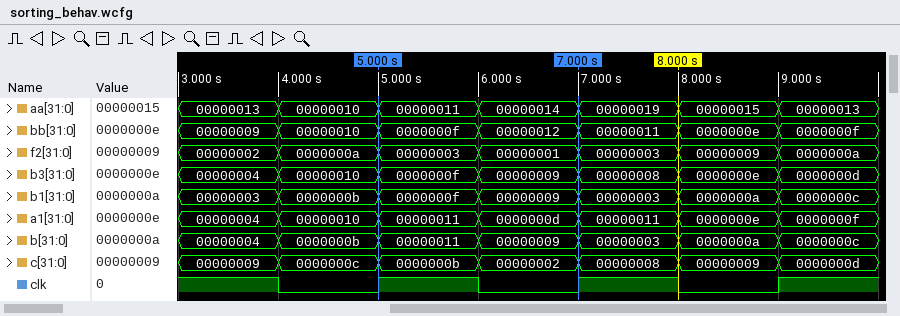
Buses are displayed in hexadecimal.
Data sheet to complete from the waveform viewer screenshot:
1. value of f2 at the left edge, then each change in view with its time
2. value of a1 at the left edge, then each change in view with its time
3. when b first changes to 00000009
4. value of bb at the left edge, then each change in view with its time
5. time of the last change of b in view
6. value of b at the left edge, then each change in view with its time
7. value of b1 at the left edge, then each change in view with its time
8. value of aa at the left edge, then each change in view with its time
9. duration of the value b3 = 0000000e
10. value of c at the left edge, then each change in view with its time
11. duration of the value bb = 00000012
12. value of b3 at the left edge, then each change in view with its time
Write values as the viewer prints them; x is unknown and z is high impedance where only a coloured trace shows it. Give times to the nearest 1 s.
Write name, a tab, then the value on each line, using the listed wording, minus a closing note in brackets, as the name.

value of f2 at the left edge, then each change in view with its time	00000002, 0000000a at 4 s, 00000003 at 5 s, 00000001 at 6 s, 00000003 at 7 s, 00000009 at 8 s, 0000000a at 9 s
value of a1 at the left edge, then each change in view with its time	00000004, 00000010 at 4 s, 00000011 at 5 s, 0000000d at 6 s, 00000011 at 7 s, 0000000e at 8 s, 0000000f at 9 s
when b first changes to 00000009	6 s
value of bb at the left edge, then each change in view with its time	00000009, 00000010 at 4 s, 0000000f at 5 s, 00000012 at 6 s, 00000011 at 7 s, 0000000e at 8 s, 0000000f at 9 s
time of the last change of b in view	9 s
value of b at the left edge, then each change in view with its time	00000004, 0000000b at 4 s, 00000011 at 5 s, 00000009 at 6 s, 00000003 at 7 s, 0000000a at 8 s, 0000000c at 9 s
value of b1 at the left edge, then each change in view with its time	00000003, 0000000b at 4 s, 0000000f at 5 s, 00000009 at 6 s, 00000003 at 7 s, 0000000a at 8 s, 0000000c at 9 s
value of aa at the left edge, then each change in view with its time	00000013, 00000010 at 4 s, 00000011 at 5 s, 00000014 at 6 s, 00000019 at 7 s, 00000015 at 8 s, 00000013 at 9 s
duration of the value b3 = 0000000e	1 s
value of c at the left edge, then each change in view with its time	00000009, 0000000c at 4 s, 0000000b at 5 s, 00000002 at 6 s, 00000008 at 7 s, 00000009 at 8 s, 0000000d at 9 s
duration of the value bb = 00000012	1 s
value of b3 at the left edge, then each change in view with its time	00000004, 00000010 at 4 s, 0000000f at 5 s, 00000009 at 6 s, 00000008 at 7 s, 0000000e at 8 s, 0000000d at 9 s
